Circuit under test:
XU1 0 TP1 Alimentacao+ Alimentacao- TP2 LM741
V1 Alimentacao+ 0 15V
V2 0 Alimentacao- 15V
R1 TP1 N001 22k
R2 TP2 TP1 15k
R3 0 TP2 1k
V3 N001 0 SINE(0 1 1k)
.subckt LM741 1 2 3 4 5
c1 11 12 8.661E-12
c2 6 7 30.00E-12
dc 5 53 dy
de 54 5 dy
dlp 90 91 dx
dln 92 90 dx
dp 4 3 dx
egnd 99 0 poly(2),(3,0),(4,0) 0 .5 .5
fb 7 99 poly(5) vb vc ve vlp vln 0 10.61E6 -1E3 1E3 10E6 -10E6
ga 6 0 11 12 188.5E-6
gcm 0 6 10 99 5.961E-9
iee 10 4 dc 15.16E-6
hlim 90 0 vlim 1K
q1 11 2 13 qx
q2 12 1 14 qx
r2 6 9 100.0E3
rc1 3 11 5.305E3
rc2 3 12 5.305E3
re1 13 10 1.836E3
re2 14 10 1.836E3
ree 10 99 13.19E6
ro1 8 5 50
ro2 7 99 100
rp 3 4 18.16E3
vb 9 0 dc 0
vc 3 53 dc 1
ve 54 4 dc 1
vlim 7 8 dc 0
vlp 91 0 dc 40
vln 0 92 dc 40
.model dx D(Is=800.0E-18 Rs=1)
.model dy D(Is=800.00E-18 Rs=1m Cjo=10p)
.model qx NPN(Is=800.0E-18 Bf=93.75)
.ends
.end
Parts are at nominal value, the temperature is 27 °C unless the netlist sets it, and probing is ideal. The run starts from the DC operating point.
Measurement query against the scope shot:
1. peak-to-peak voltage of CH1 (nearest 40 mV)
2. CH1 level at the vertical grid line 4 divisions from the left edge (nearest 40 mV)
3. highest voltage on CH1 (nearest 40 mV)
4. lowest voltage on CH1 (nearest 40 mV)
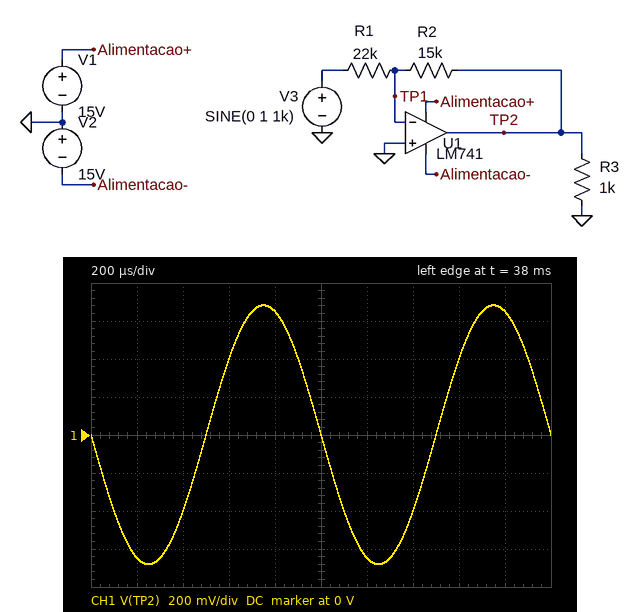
1.36 V
640 mV
680 mV
-680 mV
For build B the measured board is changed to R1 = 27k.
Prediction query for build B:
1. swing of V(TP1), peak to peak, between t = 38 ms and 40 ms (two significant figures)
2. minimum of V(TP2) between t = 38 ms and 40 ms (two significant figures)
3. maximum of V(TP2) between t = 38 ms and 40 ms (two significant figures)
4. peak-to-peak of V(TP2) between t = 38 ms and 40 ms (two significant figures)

1.2 mV
-550 mV
560 mV
1.1 V
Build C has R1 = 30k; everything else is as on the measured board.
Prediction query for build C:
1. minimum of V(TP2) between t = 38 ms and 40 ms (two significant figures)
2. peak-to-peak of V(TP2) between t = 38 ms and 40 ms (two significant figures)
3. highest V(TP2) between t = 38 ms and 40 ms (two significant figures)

-500 mV
1.0 V
500 mV
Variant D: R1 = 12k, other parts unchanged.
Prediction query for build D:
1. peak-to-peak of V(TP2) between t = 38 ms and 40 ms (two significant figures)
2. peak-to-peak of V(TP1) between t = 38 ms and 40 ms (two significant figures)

2.5 V
2.6 mV
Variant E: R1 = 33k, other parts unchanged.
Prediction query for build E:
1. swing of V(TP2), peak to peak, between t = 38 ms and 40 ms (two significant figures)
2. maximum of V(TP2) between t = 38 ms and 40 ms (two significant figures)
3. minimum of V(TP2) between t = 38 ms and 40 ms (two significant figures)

910 mV
460 mV
-450 mV
